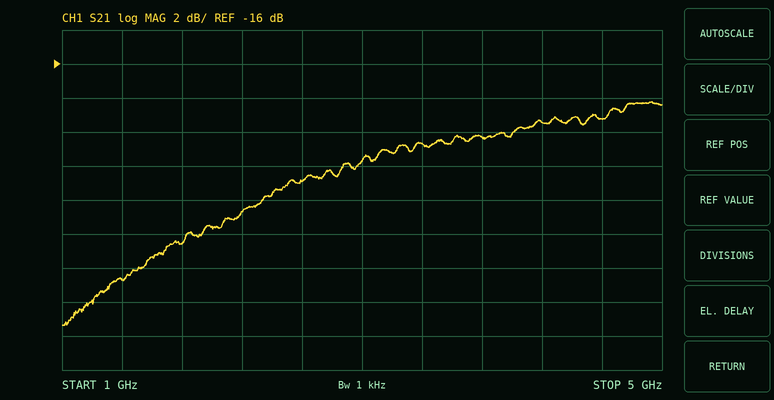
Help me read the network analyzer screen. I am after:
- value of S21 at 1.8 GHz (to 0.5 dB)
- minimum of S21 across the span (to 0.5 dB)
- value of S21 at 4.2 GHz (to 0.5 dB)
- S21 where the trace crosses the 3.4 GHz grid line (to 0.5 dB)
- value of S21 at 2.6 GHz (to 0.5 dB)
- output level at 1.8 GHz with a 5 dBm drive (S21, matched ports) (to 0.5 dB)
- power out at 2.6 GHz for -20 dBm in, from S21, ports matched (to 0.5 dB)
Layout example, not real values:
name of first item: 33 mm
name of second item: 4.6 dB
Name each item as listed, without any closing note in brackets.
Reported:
value of S21 at 1.8 GHz: -26.5 dB
minimum of S21 across the span: -31.5 dB
value of S21 at 4.2 GHz: -19.5 dB
S21 where the trace crosses the 3.4 GHz grid line: -20.5 dB
value of S21 at 2.6 GHz: -23.0 dB
output level at 1.8 GHz with a 5 dBm drive (S21, matched ports): -21.5 dBm
power out at 2.6 GHz for -20 dBm in, from S21, ports matched: -43.0 dBm
